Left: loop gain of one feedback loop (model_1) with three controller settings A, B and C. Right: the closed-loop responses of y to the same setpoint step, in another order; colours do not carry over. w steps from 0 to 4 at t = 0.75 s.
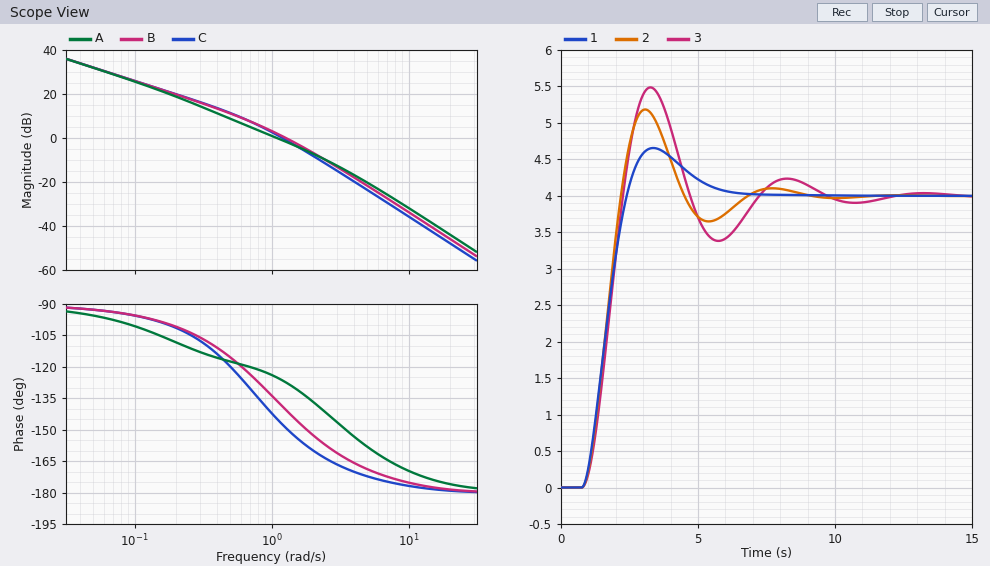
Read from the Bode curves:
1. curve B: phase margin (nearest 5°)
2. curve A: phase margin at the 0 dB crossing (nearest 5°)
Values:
40°
55°
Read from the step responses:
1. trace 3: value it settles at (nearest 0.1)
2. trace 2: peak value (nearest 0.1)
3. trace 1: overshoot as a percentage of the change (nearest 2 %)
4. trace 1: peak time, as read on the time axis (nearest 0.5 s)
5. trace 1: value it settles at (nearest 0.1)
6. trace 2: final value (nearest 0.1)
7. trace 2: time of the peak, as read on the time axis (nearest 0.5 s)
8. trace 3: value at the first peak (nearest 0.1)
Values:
4.0
5.2
16 %
3.5 s
4.0
4.0
3.0 s
5.5
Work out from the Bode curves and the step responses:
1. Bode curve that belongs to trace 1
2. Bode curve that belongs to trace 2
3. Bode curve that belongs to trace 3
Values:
A
B
C
